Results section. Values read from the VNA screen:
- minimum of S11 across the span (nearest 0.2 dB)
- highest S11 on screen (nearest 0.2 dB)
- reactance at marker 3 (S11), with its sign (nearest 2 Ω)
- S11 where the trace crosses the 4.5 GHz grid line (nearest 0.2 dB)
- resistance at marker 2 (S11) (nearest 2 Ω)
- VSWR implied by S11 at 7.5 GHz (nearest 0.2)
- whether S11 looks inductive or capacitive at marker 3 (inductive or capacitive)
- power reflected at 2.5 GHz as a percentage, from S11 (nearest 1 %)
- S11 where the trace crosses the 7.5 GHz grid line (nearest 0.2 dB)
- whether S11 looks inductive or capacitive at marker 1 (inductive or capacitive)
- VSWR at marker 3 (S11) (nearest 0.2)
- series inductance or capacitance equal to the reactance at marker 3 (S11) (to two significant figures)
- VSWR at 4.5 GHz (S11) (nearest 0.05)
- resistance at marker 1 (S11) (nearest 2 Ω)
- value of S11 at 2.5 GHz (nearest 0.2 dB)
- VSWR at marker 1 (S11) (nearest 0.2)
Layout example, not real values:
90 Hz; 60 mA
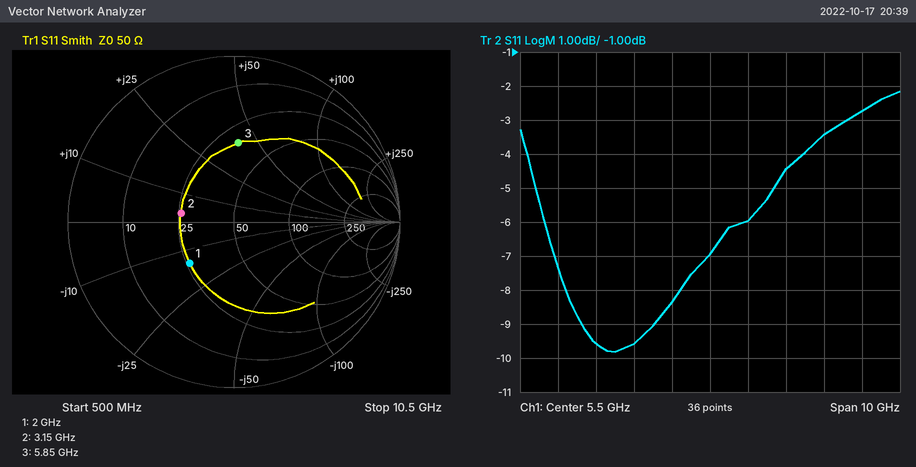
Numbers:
-9.8 dB; -2.2 dB; +40 Ω; -8.4 dB; 26 Ω; 4.0; inductive; 11 %; -4.4 dB; capacitive; 2.8; 1.1 nH; 2.25; 26 Ω; -9.6 dB; 2.2
